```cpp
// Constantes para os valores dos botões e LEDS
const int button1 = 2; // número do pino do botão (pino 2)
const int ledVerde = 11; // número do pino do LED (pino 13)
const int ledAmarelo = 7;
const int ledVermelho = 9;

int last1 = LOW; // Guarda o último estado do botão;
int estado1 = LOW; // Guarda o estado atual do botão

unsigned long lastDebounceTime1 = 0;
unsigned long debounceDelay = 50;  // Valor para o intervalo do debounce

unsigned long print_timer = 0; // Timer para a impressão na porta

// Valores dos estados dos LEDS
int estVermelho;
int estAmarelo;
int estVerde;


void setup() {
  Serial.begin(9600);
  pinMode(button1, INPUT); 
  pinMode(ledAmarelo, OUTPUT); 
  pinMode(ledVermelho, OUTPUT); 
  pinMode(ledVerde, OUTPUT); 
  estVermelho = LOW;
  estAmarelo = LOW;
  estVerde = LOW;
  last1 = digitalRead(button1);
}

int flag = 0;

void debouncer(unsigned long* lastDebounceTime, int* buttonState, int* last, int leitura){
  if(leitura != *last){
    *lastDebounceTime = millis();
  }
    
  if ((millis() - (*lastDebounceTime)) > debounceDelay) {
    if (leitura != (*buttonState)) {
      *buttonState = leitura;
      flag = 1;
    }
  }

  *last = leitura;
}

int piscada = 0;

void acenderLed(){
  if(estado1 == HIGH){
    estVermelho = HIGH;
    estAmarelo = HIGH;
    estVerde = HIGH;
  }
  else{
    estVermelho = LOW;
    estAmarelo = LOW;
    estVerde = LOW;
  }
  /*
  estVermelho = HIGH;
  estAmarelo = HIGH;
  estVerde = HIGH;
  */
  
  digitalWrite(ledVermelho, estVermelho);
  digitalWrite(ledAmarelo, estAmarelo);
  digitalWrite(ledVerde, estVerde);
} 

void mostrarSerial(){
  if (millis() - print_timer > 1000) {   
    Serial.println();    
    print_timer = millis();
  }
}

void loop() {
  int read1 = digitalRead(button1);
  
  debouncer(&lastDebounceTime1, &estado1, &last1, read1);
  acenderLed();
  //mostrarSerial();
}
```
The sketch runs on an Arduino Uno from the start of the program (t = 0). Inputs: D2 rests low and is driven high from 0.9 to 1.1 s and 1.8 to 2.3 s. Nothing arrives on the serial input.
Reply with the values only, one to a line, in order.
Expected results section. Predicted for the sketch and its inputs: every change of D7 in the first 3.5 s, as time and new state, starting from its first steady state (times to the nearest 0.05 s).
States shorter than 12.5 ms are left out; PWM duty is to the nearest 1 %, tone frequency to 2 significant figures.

0 s low; 0.95 s high; 1.15 s low; 1.85 s high; 2.35 s low
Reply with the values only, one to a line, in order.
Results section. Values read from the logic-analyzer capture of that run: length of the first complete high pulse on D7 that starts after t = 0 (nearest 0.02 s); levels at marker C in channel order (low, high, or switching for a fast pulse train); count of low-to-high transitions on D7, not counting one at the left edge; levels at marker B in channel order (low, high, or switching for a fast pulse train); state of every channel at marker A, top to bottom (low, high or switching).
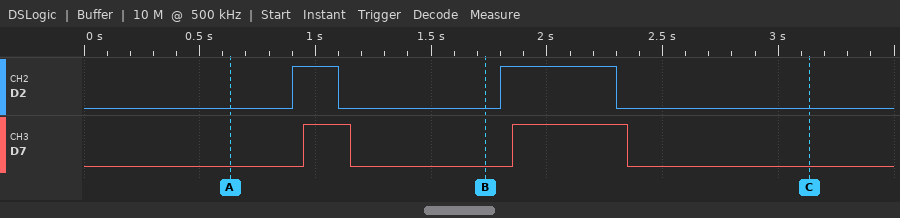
0.20 s
D2 low, D7 low
2
D2 low, D7 low
D2 low, D7 low
